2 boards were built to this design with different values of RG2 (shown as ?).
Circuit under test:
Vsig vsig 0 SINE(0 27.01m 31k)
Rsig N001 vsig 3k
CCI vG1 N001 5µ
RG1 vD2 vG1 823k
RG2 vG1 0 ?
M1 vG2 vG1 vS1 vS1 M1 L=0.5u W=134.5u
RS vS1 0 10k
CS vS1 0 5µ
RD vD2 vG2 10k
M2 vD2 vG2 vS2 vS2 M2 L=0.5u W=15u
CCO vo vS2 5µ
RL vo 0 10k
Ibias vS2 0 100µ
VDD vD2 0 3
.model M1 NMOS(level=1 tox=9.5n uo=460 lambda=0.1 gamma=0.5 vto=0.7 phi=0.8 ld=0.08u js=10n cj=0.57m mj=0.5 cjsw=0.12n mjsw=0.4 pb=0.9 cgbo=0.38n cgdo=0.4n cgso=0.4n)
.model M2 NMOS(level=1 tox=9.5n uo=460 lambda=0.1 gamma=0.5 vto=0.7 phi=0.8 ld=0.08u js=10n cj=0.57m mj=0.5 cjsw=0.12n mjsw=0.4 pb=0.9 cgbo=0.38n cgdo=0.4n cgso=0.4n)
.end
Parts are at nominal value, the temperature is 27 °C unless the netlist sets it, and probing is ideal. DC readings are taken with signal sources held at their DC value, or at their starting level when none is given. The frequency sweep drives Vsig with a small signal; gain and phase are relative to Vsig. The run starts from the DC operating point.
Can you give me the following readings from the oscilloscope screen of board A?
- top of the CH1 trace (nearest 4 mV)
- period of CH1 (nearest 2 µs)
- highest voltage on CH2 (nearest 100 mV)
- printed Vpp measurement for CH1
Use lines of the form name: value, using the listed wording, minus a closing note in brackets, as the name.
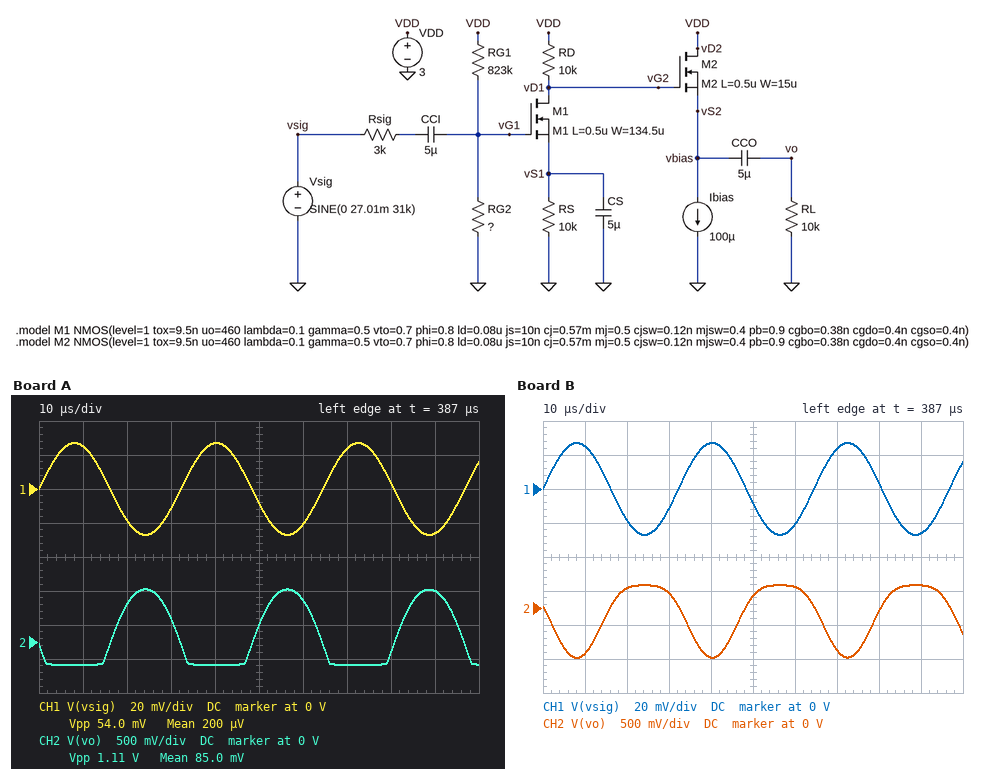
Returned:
top of the CH1 trace: 28 mV
period of CH1: 32 µs
highest voltage on CH2: 800 mV
printed Vpp measurement for CH1: 54.0 mV
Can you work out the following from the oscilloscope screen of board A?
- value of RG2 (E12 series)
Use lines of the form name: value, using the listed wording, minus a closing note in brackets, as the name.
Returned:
value of RG2: 1.8 MΩ
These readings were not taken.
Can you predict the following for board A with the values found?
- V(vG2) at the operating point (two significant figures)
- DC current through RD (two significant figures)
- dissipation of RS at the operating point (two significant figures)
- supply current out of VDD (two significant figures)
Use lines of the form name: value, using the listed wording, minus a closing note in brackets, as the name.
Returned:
V(vG2) at the operating point: 1.7 V
DC current through RD: 130 µA
dissipation of RS at the operating point: 170 µW
supply current out of VDD: 230 µA
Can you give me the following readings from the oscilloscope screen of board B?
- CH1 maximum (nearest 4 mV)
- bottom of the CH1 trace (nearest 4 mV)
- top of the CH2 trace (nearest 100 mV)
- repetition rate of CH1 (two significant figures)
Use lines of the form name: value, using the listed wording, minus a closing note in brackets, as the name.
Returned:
CH1 maximum: 28 mV
bottom of the CH1 trace: -28 mV
top of the CH2 trace: 300 mV
repetition rate of CH1: 31 kHz
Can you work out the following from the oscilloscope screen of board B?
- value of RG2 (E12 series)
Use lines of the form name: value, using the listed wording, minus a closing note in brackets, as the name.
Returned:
value of RG2: 470 kΩ
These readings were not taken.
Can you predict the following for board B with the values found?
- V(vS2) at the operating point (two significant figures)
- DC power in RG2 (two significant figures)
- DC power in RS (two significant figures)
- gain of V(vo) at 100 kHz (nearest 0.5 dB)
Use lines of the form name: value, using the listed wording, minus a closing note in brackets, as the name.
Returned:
V(vS2) at the operating point: 1.8 V
DC power in RG2: 2.5 µW
DC power in RS: 13 µW
gain of V(vo) at 100 kHz: 26.5 dB
